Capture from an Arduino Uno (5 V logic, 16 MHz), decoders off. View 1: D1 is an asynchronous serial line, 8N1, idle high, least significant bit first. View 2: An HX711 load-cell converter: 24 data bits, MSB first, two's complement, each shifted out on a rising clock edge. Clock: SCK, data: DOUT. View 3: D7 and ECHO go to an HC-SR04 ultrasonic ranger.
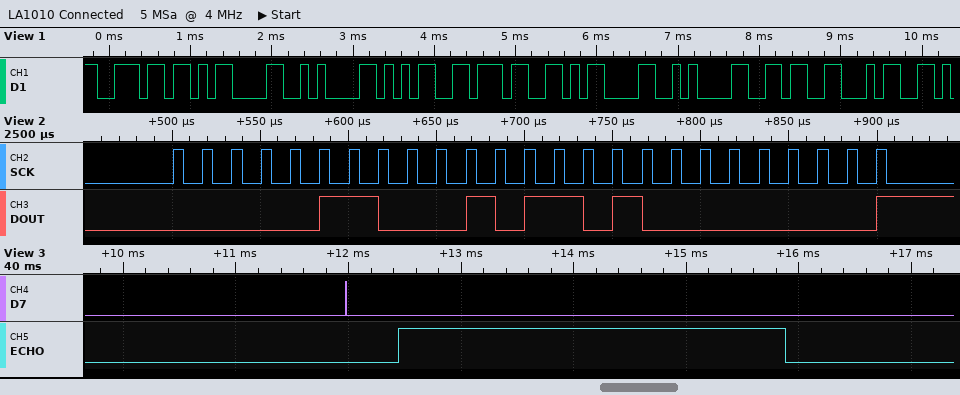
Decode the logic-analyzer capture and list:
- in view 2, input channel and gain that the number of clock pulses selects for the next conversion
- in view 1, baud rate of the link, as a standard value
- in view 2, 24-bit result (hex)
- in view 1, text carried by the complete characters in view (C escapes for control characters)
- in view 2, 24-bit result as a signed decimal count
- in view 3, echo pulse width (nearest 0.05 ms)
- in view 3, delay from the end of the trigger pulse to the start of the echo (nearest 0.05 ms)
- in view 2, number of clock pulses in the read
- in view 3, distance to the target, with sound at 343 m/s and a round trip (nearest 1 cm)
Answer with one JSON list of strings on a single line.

["channel A, gain 128", "9600 baud", "0x062D00", "\"n\\r\\n57\\r\\n64\"", "404736", "3.45 ms", "0.45 ms", "25", "59 cm"]
